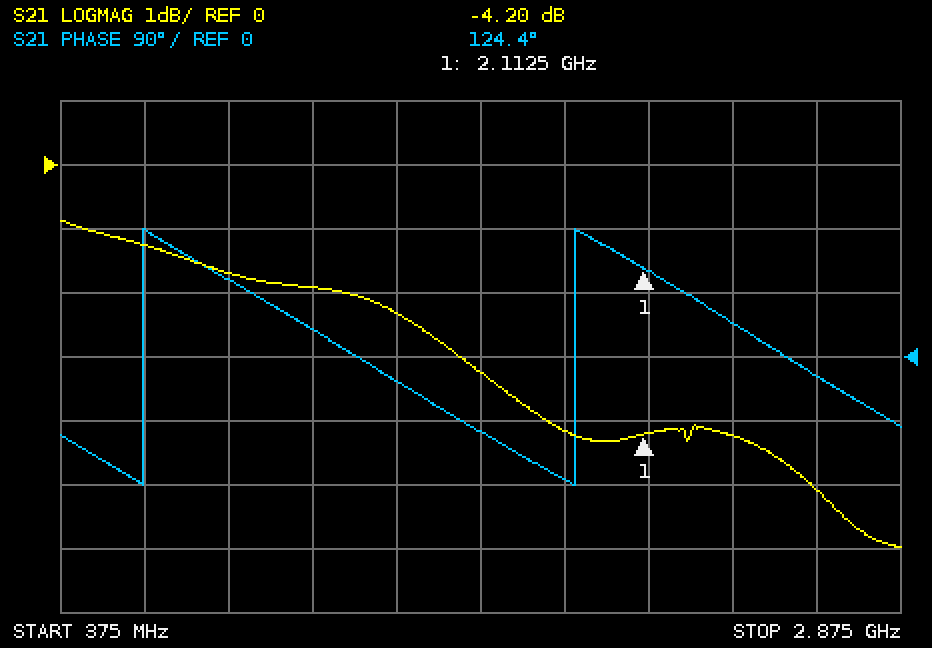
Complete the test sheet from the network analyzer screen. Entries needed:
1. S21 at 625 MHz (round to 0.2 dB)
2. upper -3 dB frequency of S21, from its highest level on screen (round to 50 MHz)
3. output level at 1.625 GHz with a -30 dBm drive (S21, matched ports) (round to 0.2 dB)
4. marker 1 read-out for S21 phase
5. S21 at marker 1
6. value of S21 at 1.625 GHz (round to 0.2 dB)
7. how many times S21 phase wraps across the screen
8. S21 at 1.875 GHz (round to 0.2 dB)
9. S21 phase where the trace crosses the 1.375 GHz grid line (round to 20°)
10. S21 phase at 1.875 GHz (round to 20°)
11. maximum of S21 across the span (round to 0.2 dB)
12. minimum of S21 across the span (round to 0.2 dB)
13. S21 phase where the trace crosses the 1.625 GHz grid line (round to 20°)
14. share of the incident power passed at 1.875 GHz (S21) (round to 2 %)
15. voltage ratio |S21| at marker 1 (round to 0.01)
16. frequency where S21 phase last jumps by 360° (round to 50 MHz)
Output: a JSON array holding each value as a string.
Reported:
["-1.2 dB", "1.80 GHz", "-33.2 dBm", "124.4°", "-4.20 dB", "-3.2 dB", "2", "-4.2 dB", "-40°", "-180°", "-0.8 dB", "-6.0 dB", "-100°", "38 %", "0.62", "1.90 GHz"]
